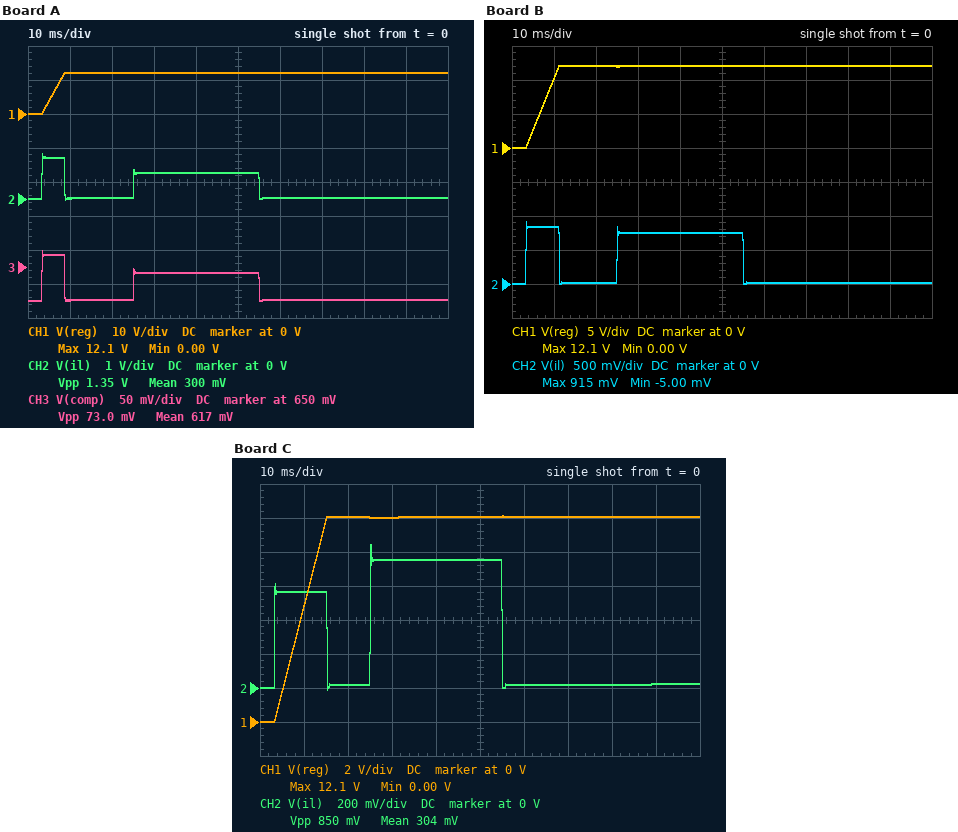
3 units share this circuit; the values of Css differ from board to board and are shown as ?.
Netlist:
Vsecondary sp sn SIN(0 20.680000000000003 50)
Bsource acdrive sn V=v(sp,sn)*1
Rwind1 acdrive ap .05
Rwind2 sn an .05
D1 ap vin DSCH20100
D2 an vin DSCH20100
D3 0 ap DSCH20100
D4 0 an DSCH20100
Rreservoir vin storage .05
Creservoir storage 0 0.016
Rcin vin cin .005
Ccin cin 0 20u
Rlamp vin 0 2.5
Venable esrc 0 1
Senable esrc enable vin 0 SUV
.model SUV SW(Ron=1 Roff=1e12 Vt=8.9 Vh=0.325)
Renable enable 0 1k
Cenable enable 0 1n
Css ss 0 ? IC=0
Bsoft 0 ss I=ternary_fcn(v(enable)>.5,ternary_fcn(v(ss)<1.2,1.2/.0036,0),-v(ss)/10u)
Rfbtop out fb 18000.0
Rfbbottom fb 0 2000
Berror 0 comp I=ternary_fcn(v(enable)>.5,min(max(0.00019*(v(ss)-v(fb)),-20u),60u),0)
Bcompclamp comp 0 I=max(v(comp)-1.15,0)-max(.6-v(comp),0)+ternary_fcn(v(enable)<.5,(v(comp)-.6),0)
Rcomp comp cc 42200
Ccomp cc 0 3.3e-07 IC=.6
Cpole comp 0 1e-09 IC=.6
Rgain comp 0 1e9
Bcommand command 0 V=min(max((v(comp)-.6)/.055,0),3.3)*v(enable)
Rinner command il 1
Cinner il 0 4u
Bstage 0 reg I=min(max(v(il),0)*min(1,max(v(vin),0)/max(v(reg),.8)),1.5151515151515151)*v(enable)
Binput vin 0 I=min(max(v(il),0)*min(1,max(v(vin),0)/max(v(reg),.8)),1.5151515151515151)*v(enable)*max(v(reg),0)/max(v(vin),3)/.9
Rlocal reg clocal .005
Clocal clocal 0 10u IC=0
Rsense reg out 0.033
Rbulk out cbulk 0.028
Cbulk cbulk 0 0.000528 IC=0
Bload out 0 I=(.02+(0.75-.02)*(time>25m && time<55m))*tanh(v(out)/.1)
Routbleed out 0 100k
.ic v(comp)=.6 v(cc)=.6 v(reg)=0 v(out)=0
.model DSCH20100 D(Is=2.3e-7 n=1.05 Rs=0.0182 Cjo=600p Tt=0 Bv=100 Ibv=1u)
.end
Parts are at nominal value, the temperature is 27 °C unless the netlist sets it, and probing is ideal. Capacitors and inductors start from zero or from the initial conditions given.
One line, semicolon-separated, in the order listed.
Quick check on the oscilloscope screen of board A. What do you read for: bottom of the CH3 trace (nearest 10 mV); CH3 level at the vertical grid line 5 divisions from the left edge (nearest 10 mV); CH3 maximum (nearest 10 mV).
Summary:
600 mV; 640 mV; 670 mV
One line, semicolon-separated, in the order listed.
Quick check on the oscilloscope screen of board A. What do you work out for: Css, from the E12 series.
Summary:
1.5 F
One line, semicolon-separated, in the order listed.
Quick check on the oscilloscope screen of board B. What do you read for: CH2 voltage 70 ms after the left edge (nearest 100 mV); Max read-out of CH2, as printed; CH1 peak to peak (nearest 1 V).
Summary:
0 V; 915 mV; 12 V
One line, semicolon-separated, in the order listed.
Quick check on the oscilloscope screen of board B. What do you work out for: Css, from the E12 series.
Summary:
2.2 F
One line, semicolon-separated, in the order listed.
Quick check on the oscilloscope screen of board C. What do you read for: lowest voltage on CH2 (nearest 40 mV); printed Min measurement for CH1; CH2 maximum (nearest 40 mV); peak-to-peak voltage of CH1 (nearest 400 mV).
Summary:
0 V; 0.00 V; 840 mV; 12.0 V
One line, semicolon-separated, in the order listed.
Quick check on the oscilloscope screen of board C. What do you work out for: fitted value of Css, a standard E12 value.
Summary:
3.3 F
